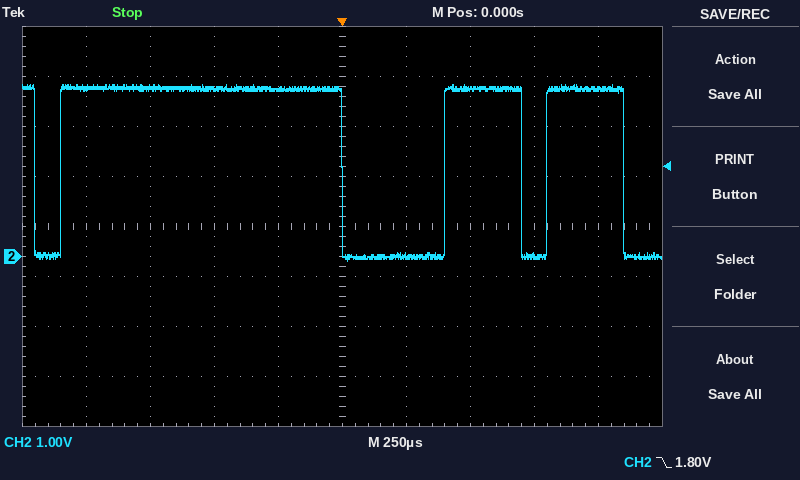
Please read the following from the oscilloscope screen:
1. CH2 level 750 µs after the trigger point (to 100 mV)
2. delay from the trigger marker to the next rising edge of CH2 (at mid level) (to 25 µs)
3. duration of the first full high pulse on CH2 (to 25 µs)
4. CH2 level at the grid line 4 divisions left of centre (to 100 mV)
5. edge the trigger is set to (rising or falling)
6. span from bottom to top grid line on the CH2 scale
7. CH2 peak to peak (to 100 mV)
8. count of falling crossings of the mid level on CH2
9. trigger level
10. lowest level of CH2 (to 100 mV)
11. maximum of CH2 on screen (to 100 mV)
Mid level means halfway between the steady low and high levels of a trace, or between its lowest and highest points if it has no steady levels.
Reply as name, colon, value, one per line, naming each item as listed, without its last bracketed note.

CH2 level 750 µs after the trigger point: 0.0 V
delay from the trigger marker to the next rising edge of CH2 (at mid level): 400 µs
duration of the first full high pulse on CH2: 1.100 ms
CH2 level at the grid line 4 divisions left of centre: 3.4 V
edge the trigger is set to: falling
span from bottom to top grid line on the CH2 scale: 8 V
CH2 peak to peak: 3.5 V
count of falling crossings of the mid level on CH2: 4
trigger level: 1.80 V
lowest level of CH2: -100 mV
maximum of CH2 on screen: 3.4 V
